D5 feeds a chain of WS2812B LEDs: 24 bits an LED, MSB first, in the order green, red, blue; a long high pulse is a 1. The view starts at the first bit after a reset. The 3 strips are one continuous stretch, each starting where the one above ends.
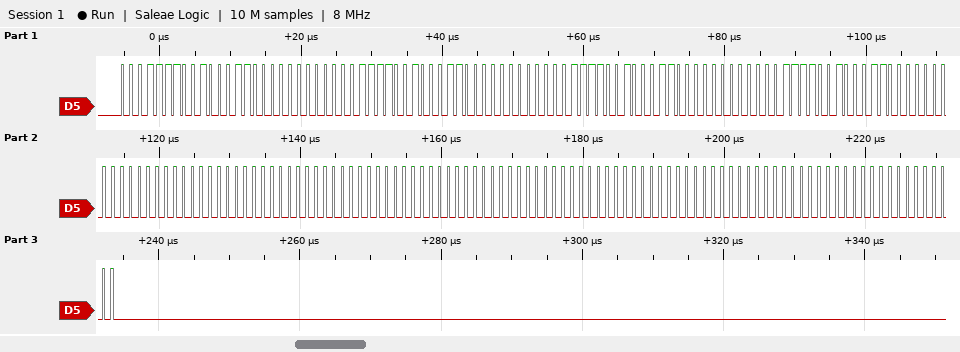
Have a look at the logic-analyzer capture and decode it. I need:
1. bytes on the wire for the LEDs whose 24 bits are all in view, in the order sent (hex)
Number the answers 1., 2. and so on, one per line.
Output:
1. 1E 46 00 1E 46 00 1E 46 00 1E 46 00 00 00 00 00 00 00 00 00 00 00 00 00
